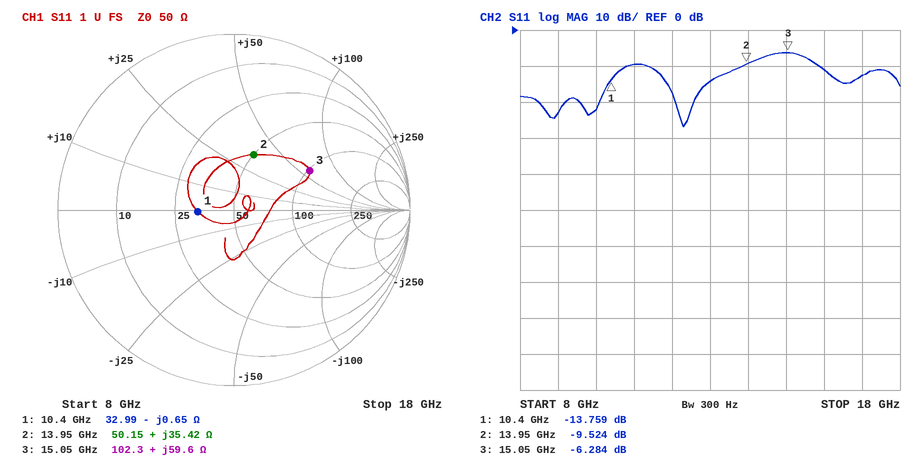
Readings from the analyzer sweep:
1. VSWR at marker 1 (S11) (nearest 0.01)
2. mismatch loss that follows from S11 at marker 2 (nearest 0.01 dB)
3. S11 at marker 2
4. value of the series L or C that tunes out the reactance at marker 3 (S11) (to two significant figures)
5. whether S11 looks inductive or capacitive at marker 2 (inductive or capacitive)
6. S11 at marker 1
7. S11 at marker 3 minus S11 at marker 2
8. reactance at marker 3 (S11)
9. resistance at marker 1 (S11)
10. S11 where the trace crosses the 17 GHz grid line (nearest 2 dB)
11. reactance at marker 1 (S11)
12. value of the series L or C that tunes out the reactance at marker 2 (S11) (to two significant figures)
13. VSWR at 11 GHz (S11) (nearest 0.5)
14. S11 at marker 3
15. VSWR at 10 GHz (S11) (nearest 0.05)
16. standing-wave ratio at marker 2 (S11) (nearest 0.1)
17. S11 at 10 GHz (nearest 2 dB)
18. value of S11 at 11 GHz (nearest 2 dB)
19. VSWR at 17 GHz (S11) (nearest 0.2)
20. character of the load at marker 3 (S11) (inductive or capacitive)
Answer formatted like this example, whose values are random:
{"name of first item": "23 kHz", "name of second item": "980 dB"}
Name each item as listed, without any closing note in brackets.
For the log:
{"VSWR at marker 1 (S11)": "1.52", "mismatch loss that follows from S11 at marker 2": "0.51 dB", "S11 at marker 2": "-9.524 dB", "value of the series L or C that tunes out the reactance at marker 3 (S11)": "180 fF", "whether S11 looks inductive or capacitive at marker 2": "inductive", "S11 at marker 1": "-13.759 dB", "S11 at marker 3 minus S11 at marker 2": "3.240 dB", "reactance at marker 3": "+59.6 Ω", "resistance at marker 1": "32.99 Ω", "S11 where the trace crosses the 17 GHz grid line": "-12 dB", "reactance at marker 1": "-0.65 Ω", "value of the series L or C that tunes out the reactance at marker 2 (S11)": "320 fF", "VSWR at 11 GHz (S11)": "2.0", "S11 at marker 3": "-6.284 dB", "VSWR at 10 GHz (S11)": "1.15", "standing-wave ratio at marker 2 (S11)": "2.0", "S11 at 10 GHz": "-22 dB", "value of S11 at 11 GHz": "-10 dB", "VSWR at 17 GHz (S11)": "1.6", "character of the load at marker 3 (S11)": "inductive"}
